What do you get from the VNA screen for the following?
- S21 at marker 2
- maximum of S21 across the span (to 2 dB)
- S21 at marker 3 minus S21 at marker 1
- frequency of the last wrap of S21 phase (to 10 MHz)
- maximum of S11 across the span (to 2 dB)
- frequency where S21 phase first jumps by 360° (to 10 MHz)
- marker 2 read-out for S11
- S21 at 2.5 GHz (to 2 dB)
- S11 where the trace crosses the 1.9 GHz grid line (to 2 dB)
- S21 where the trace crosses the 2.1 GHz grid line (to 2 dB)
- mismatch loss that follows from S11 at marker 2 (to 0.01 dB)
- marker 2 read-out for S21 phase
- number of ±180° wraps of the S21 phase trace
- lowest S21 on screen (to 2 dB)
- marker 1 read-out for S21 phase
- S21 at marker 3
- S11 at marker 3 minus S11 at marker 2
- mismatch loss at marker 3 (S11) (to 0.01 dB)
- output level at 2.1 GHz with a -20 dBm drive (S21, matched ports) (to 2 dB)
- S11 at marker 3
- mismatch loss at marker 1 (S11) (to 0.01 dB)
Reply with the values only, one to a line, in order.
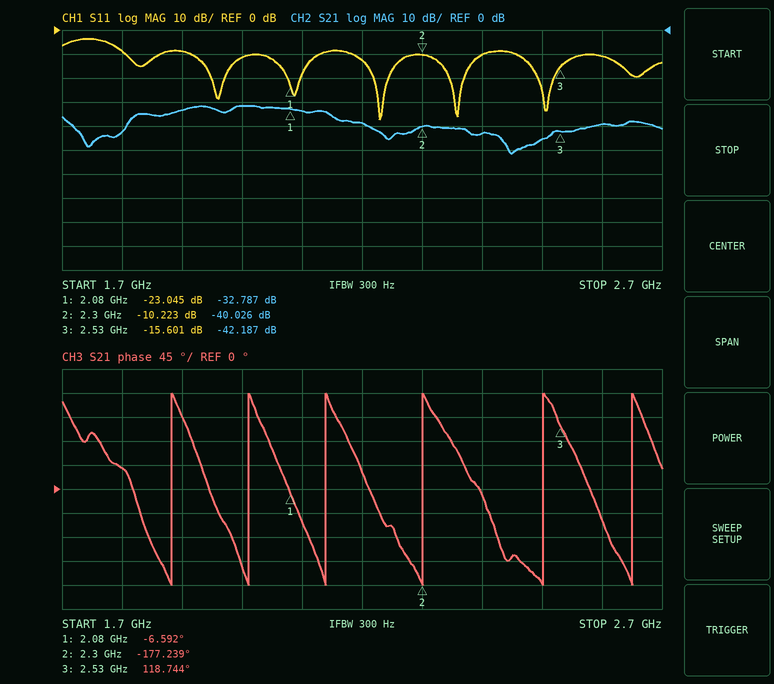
-40.026 dB
-32 dB
-9.400 dB
2.65 GHz
-4 dB
1.88 GHz
-10.223 dB
-46 dB
-8 dB
-34 dB
0.43 dB
-177.239°
6
-52 dB
-6.592°
-42.187 dB
-5.378 dB
0.12 dB
-54 dBm
-15.601 dB
0.02 dB
